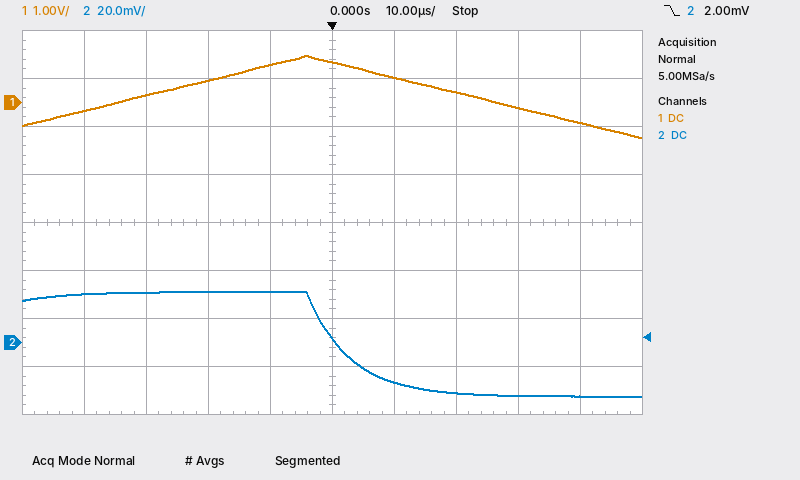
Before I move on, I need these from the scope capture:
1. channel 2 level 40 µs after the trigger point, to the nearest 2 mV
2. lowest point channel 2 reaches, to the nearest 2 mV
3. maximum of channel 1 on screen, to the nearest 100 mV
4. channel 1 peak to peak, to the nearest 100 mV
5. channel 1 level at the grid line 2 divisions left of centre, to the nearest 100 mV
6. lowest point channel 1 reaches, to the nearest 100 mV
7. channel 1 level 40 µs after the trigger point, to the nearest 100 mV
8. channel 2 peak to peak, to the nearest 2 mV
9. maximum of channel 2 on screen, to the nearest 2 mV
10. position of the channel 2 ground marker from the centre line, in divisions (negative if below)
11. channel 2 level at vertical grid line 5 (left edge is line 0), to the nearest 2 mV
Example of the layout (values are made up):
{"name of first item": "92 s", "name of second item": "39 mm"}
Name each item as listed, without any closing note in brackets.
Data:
{"channel 2 level 40 µs after the trigger point, to the nearest 2 mV": "-22 mV", "lowest point channel 2 reaches, to the nearest 2 mV": "-22 mV", "maximum of channel 1 on screen, to the nearest 100 mV": "1.0 V", "channel 1 peak to peak, to the nearest 100 mV": "1.7 V", "channel 1 level at the grid line 2 divisions left of centre, to the nearest 100 mV": "500 mV", "lowest point channel 1 reaches, to the nearest 100 mV": "-700 mV", "channel 1 level 40 µs after the trigger point, to the nearest 100 mV": "-400 mV", "channel 2 peak to peak, to the nearest 2 mV": "44 mV", "maximum of channel 2 on screen, to the nearest 2 mV": "22 mV", "position of the channel 2 ground marker from the centre line, in divisions": "-2.5 div", "channel 2 level at vertical grid line 5 (left edge is line 0), to the nearest 2 mV": "2 mV"}
